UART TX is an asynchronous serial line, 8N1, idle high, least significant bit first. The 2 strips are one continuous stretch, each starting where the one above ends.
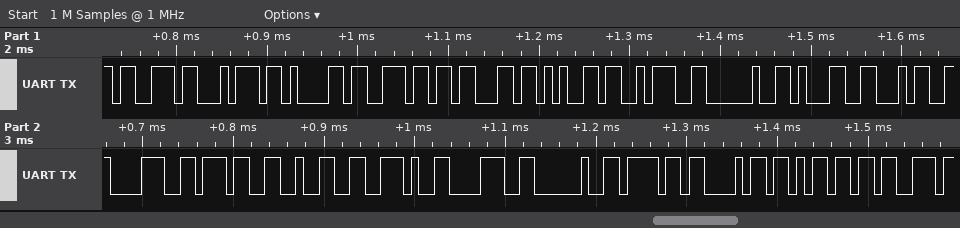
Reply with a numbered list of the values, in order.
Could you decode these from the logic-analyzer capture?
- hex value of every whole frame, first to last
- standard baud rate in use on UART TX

1. 73 74 61 6E 63 65 3A 20 31 34 38 37 32 2E 38 20 6F 68 6D 73
2. 115200 baud
